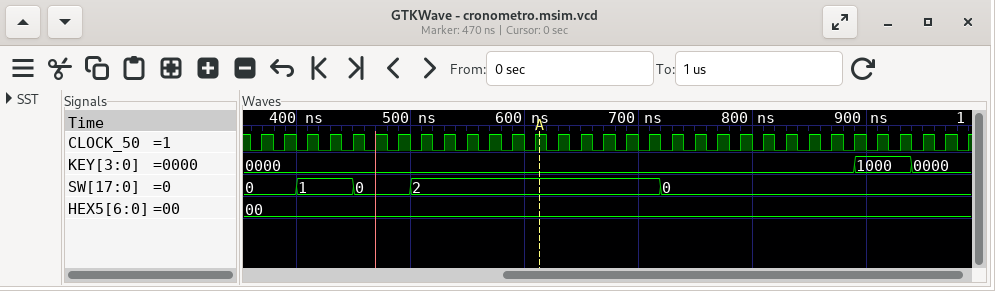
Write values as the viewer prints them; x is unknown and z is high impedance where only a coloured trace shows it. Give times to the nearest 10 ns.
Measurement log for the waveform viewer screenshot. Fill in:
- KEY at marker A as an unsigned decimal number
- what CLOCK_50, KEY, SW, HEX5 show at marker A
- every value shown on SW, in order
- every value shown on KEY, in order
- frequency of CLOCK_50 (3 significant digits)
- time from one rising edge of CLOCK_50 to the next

0
CLOCK_50=1, KEY=0000, SW=2, HEX5=00
0, 1, 0, 2, 0
0000, 1000, 0000
50.0 MHz
20 ns
